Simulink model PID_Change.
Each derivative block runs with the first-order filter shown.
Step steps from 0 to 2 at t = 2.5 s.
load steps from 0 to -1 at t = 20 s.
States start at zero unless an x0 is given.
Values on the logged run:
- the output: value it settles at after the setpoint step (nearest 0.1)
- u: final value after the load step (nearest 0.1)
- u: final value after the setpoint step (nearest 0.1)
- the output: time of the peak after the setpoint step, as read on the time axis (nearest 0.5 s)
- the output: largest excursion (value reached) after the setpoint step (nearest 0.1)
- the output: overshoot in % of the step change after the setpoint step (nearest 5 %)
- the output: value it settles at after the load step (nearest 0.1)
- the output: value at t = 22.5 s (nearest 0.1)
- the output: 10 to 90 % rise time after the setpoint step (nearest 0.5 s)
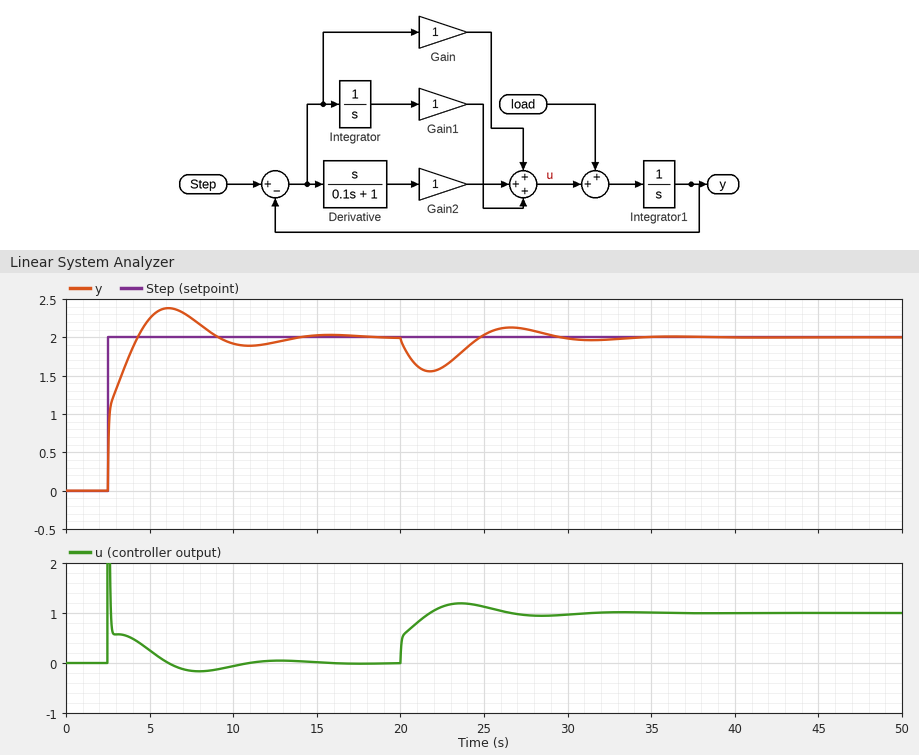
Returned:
2.0
1.0
0.0
6.0 s
2.4
20 %
2.0
1.6
1.5 s
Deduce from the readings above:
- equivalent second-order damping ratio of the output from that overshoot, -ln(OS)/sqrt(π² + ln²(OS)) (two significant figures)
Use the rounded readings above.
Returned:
0.46
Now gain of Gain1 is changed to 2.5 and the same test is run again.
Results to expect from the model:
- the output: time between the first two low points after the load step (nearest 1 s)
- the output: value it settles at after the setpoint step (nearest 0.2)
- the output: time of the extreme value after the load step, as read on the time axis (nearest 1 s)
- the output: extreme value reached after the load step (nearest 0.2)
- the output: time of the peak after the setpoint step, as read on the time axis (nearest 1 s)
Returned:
6 s
2.0
21 s
1.6
5 s
